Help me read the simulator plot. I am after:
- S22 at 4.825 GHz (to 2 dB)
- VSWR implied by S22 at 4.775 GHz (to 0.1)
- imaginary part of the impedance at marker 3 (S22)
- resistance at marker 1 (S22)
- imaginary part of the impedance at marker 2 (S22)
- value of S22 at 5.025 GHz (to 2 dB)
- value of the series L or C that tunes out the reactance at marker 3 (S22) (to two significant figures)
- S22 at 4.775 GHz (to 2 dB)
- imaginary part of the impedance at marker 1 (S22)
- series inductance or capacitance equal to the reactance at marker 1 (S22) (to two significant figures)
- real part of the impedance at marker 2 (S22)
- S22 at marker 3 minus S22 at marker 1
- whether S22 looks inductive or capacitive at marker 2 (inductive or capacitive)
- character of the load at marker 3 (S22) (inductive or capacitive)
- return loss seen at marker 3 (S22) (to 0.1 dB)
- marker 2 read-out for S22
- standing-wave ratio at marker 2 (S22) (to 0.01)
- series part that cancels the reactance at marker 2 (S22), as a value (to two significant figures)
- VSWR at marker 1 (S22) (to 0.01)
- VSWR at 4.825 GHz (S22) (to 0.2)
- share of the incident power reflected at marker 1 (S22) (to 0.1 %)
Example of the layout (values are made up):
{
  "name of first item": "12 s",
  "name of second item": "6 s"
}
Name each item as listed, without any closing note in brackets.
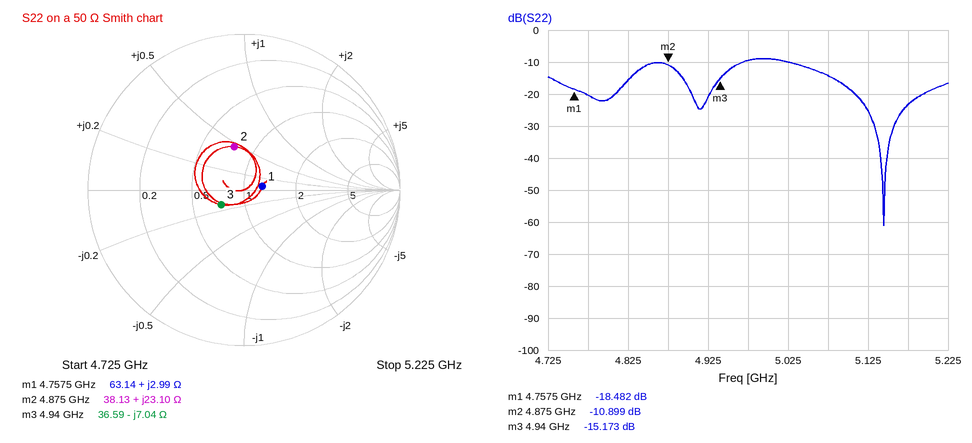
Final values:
{
  "S22 at 4.825 GHz": "-16 dB",
  "VSWR implied by S22 at 4.775 GHz": "1.2",
  "imaginary part of the impedance at marker 3": "-7.04 Ω",
  "resistance at marker 1": "63.14 Ω",
  "imaginary part of the impedance at marker 2": "+23.10 Ω",
  "value of S22 at 5.025 GHz": "-10 dB",
  "value of the series L or C that tunes out the reactance at marker 3 (S22)": "230 pH",
  "S22 at 4.775 GHz": "-20 dB",
  "imaginary part of the impedance at marker 1": "+2.99 Ω",
  "series inductance or capacitance equal to the reactance at marker 1 (S22)": "100 pH",
  "real part of the impedance at marker 2": "38.13 Ω",
  "S22 at marker 3 minus S22 at marker 1": "3.309 dB",
  "whether S22 looks inductive or capacitive at marker 2": "inductive",
  "character of the load at marker 3 (S22)": "capacitive",
  "return loss seen at marker 3 (S22)": "15.2 dB",
  "marker 2 read-out for S22": "-10.899 dB",
  "standing-wave ratio at marker 2 (S22)": "1.80",
  "series part that cancels the reactance at marker 2 (S22), as a value": "1.4 pF",
  "VSWR at marker 1 (S22)": "1.27",
  "VSWR at 4.825 GHz (S22)": "1.4",
  "share of the incident power reflected at marker 1 (S22)": "1.4 %"
}
